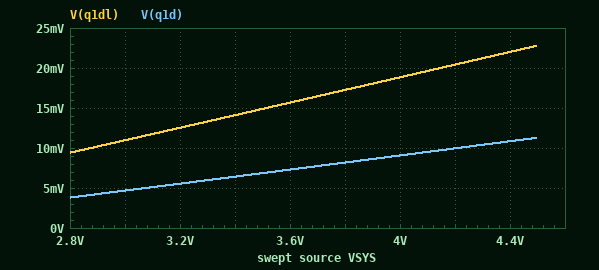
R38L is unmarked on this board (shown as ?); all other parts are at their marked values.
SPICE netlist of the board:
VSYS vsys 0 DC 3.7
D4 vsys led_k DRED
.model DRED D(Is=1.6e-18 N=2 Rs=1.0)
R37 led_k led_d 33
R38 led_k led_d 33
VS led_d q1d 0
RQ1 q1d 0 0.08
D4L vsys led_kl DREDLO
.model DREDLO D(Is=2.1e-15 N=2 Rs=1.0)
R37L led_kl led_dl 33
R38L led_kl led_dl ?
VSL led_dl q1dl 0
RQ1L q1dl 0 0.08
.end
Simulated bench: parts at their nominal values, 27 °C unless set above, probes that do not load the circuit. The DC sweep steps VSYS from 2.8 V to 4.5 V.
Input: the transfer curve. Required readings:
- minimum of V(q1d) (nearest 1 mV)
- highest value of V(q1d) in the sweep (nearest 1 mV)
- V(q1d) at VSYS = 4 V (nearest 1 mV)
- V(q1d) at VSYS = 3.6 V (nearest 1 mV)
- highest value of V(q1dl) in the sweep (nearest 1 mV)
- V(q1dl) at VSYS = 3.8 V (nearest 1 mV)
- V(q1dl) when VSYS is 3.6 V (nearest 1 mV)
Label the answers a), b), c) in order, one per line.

a) 4 mV
b) 11 mV
c) 9 mV
d) 7 mV
e) 23 mV
f) 17 mV
g) 16 mV
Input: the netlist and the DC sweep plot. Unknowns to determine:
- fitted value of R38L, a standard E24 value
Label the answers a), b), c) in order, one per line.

a) 12 Ω
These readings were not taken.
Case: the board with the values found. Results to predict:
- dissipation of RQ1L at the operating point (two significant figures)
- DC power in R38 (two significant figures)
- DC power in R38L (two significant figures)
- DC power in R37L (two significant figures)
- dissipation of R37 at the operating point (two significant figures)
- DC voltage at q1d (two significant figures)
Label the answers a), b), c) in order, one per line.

a) 3.4 mW
b) 77 mW
c) 270 mW
d) 99 mW
e) 77 mW
f) 7.7 mV
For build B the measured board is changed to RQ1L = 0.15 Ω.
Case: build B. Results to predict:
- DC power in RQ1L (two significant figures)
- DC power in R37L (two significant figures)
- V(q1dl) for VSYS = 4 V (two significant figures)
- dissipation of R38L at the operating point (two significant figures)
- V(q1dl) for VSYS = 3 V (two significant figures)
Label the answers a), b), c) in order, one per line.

a) 6.3 mW
b) 98 mW
c) 35 mV
d) 270 mW
e) 20 mV
